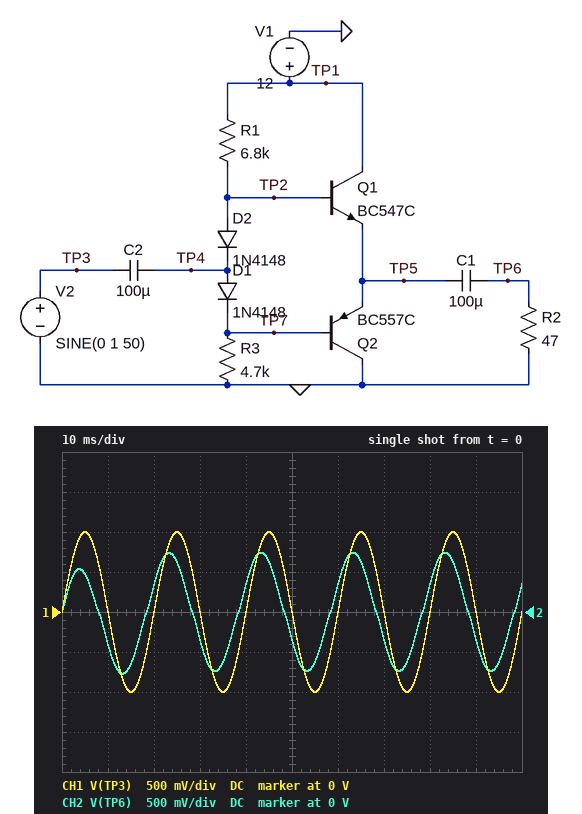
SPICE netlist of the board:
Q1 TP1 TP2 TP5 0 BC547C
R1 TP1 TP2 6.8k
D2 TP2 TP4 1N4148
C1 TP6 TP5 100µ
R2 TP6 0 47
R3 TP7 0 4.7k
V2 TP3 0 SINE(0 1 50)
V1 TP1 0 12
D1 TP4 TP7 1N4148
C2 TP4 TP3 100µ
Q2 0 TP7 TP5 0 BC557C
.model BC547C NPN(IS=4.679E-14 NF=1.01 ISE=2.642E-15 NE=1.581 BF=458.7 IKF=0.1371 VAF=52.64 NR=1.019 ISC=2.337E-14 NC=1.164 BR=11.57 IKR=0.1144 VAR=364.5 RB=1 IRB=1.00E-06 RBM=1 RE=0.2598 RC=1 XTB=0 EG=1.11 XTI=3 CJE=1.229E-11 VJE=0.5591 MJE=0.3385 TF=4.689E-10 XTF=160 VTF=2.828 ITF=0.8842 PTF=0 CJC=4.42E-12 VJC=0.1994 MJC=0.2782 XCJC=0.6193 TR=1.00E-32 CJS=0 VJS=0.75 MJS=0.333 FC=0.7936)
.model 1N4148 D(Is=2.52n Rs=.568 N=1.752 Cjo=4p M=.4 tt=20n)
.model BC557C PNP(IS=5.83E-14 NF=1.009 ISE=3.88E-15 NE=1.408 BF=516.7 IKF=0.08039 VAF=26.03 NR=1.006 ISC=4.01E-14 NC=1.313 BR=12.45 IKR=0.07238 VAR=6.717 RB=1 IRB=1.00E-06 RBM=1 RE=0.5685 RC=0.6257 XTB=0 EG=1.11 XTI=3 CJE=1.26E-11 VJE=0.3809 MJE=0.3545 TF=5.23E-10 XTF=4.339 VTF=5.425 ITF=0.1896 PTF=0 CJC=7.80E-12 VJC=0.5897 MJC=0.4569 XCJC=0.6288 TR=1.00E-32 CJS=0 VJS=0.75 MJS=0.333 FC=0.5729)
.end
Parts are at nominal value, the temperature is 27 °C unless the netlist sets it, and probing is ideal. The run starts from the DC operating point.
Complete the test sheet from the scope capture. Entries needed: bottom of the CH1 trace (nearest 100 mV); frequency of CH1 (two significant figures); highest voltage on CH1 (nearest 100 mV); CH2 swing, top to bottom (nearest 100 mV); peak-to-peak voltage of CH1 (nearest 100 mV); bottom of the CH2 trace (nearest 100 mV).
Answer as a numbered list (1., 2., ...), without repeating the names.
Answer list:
1. -1.0 V
2. 50 Hz
3. 1.0 V
4. 1.5 V
5. 2.0 V
6. -800 mV
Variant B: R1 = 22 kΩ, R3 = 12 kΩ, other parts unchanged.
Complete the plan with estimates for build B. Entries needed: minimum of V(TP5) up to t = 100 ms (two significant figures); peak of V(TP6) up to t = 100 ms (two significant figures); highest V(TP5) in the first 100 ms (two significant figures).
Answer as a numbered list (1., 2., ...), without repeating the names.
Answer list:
1. 3.6 V
2. 710 mV
3. 5.2 V
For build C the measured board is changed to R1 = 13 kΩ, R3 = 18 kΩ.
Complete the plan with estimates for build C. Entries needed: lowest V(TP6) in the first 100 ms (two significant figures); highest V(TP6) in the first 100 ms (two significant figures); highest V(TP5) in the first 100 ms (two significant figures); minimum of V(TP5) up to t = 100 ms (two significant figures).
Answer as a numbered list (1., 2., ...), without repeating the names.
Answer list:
1. -740 mV
2. 710 mV
3. 7.7 V
4. 6.0 V
